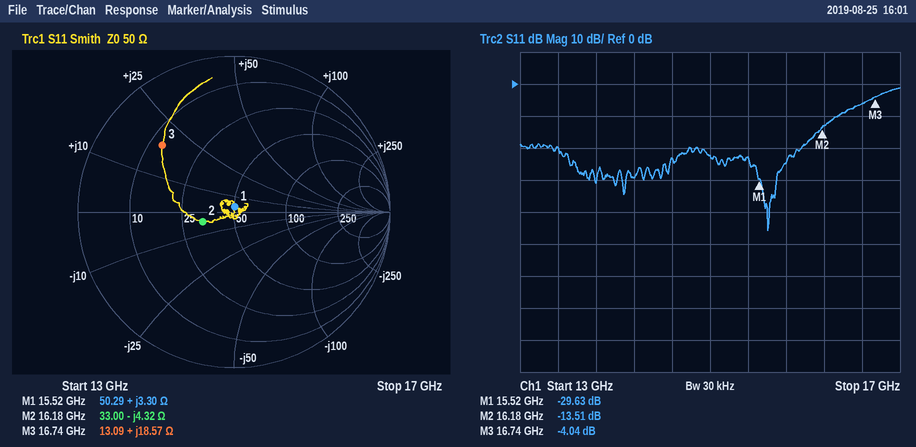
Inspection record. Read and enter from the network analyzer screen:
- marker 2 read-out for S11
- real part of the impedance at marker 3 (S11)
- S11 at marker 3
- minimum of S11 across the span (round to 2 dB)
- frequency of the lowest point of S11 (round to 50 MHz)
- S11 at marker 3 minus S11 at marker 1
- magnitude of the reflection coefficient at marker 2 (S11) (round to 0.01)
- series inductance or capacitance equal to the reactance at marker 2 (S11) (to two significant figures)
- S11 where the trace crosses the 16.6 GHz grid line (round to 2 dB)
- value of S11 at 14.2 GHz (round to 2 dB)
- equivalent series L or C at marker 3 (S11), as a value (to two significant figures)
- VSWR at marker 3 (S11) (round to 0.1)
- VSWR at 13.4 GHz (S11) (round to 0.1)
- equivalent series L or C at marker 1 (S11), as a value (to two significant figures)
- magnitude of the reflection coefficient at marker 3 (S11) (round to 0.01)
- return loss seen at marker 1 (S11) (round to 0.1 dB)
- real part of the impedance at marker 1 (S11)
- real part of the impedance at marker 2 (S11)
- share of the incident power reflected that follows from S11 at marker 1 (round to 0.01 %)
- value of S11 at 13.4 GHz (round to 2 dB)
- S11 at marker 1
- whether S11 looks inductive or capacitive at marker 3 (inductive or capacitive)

-13.51 dB
13.09 Ω
-4.04 dB
-46 dB
15.60 GHz
25.59 dB
0.21
2.3 pF
-6 dB
-30 dB
180 pH
4.4
1.2
34 pH
0.63
29.6 dB
50.29 Ω
33.00 Ω
0.11 %
-20 dB
-29.63 dB
inductive
